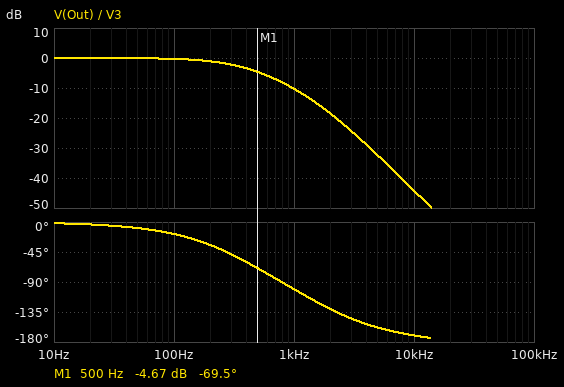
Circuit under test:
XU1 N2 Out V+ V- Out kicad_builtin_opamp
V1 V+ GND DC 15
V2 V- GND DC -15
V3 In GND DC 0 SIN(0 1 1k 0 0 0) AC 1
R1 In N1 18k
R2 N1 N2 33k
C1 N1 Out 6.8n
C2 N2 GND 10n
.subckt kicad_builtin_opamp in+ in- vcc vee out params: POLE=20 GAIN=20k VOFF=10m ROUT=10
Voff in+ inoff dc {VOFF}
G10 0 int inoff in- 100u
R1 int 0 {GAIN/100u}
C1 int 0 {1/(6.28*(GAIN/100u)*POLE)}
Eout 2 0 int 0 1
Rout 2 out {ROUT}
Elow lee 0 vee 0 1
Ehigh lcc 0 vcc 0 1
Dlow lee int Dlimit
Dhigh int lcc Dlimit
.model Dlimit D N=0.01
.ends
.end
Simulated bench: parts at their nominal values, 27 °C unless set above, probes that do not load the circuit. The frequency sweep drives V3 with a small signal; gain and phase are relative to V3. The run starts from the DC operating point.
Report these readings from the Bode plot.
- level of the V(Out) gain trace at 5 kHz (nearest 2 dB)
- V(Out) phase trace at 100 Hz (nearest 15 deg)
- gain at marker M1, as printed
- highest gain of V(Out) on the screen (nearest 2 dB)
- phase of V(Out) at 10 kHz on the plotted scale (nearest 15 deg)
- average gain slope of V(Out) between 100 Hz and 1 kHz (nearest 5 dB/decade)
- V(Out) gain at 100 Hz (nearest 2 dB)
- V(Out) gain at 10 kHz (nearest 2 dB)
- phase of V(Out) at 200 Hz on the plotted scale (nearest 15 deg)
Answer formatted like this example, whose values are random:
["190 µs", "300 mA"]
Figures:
["-32 dB", "-15 deg", "-4.67 dB", "0 dB", "-165 deg", "-10 dB/decade", "0 dB", "-44 dB", "-30 deg"]
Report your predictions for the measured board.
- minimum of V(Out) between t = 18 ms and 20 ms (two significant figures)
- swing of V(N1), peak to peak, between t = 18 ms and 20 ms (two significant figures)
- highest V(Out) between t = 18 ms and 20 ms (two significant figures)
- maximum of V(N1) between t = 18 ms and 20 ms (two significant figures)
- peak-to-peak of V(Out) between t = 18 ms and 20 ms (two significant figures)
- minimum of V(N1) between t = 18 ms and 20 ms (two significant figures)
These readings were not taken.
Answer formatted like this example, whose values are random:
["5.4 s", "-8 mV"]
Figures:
["-320 mV", "1.4 V", "300 mV", "710 mV", "610 mV", "-710 mV"]
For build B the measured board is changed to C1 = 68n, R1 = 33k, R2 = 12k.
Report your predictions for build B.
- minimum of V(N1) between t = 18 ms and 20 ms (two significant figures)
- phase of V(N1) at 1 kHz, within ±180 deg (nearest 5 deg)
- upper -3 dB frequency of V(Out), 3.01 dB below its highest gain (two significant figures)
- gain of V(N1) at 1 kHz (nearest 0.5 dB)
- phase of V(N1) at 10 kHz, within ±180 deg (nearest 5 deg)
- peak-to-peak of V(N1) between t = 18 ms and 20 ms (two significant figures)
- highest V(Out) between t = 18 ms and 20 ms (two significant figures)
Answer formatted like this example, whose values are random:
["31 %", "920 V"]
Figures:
["-120 mV", "-125 deg", "360 Hz", "-18.0 dB", "-95 deg", "250 mV", "89 mV"]
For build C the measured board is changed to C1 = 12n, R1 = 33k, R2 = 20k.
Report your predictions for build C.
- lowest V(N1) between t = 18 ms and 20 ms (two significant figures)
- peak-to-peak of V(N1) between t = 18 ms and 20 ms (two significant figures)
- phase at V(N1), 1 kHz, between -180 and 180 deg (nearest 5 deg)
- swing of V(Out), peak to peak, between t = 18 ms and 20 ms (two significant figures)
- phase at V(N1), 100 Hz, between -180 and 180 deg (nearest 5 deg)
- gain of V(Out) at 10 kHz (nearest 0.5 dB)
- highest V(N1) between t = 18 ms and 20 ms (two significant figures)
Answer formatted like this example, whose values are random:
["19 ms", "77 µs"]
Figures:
["-410 mV", "810 mV", "-70 deg", "510 mV", "-10 deg", "-50.0 dB", "410 mV"]
